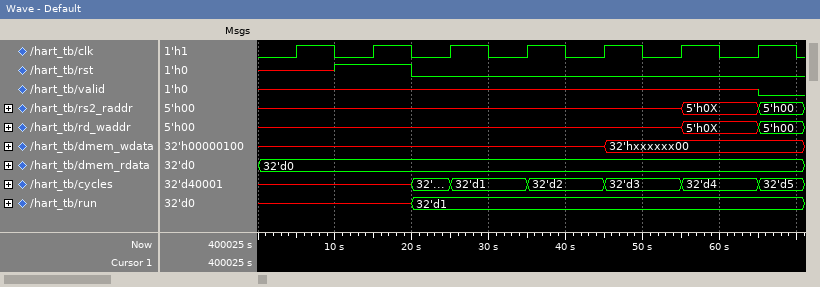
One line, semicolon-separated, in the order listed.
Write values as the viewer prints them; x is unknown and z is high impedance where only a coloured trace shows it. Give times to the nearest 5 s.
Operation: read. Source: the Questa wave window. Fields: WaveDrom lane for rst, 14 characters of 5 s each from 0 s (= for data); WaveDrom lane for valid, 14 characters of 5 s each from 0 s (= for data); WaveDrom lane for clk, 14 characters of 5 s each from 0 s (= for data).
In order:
{name: 'rst', wave: 'x.1.0.........'}; {name: 'valid', wave: 'x............0'}; {name: 'clk', wave: '01010101010101'}
